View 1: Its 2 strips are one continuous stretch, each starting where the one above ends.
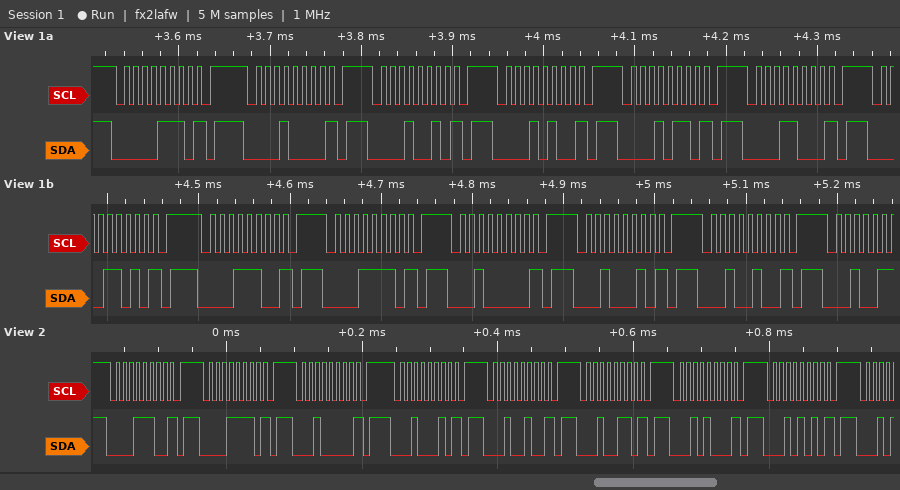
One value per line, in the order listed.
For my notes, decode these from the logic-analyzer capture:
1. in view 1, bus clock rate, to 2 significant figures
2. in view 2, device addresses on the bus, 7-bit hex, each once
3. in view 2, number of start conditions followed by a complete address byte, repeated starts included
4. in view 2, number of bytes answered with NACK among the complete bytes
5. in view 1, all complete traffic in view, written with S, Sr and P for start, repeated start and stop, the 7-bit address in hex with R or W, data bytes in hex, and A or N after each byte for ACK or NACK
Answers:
100 kHz
0x0E 0x0F 0x10 0x11 0x12 0x13 0x14 0x15
8
8
S 07W N P S 08W N P S 09W N P S 0AW N P S 0BW N P S 0CW N P S 0DW N P S 0EW N P S 0FW N P S 10W N P S 11W N P S 12W N P
